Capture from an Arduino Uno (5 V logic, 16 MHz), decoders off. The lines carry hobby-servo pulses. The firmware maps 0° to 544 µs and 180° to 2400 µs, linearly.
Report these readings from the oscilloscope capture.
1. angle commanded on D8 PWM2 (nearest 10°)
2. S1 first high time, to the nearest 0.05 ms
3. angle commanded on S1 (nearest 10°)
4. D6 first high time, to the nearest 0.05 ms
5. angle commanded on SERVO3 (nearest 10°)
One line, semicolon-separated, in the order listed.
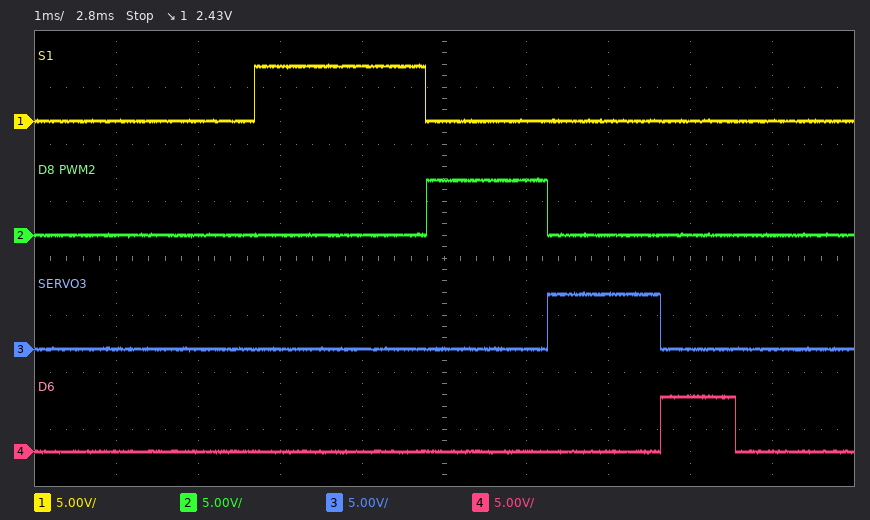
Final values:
90°; 2.10 ms; 150°; 0.90 ms; 80°
